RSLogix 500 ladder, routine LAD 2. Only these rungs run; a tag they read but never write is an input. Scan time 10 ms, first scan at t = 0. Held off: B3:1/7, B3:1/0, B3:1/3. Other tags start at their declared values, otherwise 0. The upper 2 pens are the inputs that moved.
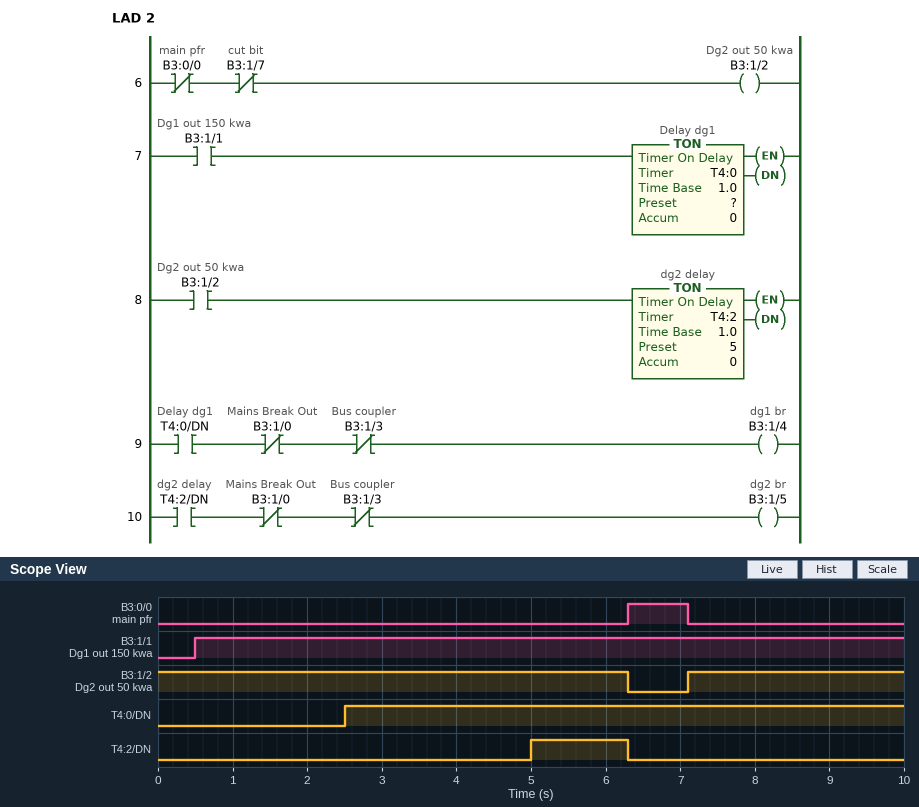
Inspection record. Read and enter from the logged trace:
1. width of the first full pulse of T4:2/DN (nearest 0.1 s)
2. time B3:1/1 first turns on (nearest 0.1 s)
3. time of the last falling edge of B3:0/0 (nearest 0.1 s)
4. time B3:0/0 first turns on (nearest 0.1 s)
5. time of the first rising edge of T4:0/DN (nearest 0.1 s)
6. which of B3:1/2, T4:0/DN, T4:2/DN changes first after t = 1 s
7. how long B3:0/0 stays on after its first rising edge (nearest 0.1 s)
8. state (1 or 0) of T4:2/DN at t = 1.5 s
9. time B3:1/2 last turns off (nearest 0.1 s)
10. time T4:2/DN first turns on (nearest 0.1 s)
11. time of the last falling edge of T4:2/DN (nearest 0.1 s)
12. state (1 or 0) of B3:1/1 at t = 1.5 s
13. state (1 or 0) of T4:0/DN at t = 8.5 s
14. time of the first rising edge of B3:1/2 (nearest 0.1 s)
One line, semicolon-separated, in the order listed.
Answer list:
1.3 s; 0.5 s; 7.1 s; 6.3 s; 2.5 s; T4:0/DN; 0.8 s; 0; 6.3 s; 5.0 s; 6.3 s; 1; 1; 7.1 s
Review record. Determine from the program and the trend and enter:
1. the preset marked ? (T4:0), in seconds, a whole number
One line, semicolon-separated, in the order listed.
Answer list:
2 s
